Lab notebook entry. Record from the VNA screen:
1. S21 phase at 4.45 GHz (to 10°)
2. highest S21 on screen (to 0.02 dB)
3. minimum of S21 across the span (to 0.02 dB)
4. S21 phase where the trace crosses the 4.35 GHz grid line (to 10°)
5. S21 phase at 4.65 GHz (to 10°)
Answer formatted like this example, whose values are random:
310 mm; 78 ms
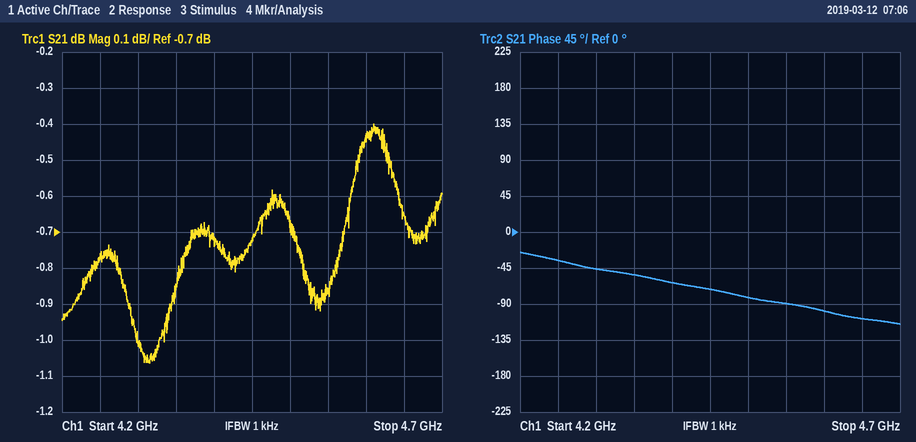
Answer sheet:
-70°; -0.40 dB; -1.06 dB; -50°; -110°
